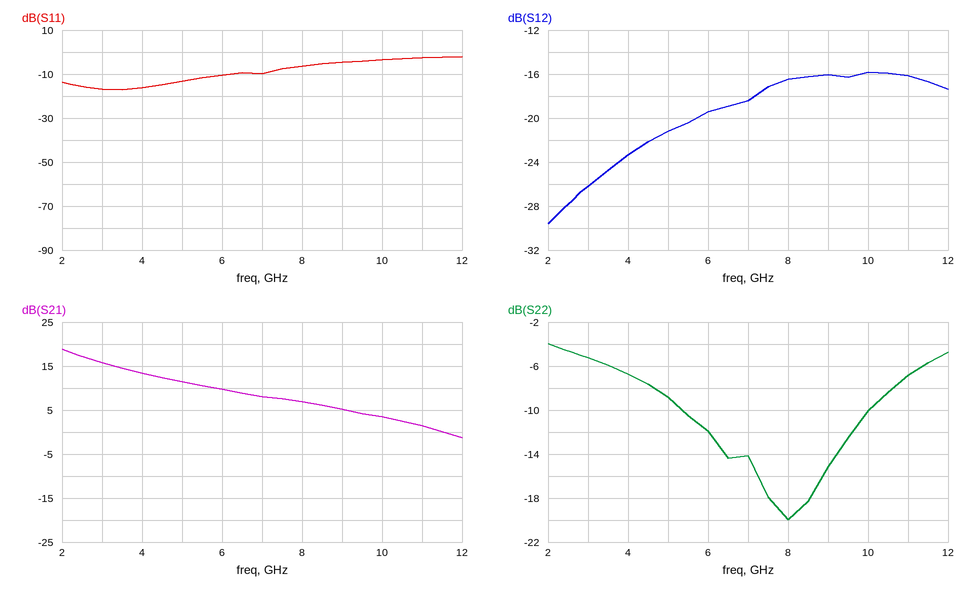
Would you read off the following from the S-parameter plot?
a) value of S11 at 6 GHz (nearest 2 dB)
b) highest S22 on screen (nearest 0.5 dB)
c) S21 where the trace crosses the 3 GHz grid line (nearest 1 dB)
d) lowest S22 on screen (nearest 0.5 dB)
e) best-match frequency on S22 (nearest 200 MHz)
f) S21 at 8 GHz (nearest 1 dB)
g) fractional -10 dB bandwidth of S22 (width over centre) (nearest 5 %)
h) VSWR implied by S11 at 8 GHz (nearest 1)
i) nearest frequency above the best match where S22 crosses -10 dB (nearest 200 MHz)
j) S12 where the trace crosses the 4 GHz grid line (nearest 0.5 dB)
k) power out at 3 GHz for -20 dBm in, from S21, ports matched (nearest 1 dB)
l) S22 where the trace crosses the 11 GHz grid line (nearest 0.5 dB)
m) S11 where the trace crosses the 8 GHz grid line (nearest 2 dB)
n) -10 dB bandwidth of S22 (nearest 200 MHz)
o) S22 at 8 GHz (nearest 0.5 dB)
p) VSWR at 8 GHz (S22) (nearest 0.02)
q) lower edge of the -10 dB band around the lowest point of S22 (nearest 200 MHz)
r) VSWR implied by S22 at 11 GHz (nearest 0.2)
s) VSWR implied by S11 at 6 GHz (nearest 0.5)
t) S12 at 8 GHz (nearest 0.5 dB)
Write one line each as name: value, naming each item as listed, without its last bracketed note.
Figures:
value of S11 at 6 GHz: -10 dB
highest S22 on screen: -4.0 dB
S21 where the trace crosses the 3 GHz grid line: 16 dB
lowest S22 on screen: -20.0 dB
best-match frequency on S22: 8.0 GHz
S21 at 8 GHz: 7 dB
fractional -10 dB bandwidth of S22 (width over centre): 60 %
VSWR implied by S11 at 8 GHz: 3
nearest frequency above the best match where S22 crosses -10 dB: 10.0 GHz
S12 where the trace crosses the 4 GHz grid line: -23.5 dB
power out at 3 GHz for -20 dBm in, from S21, ports matched: -4 dBm
S22 where the trace crosses the 11 GHz grid line: -7.0 dB
S11 where the trace crosses the 8 GHz grid line: -6 dB
-10 dB bandwidth of S22: 4.6 GHz
S22 at 8 GHz: -20.0 dB
VSWR at 8 GHz (S22): 1.22
lower edge of the -10 dB band around the lowest point of S22: 5.4 GHz
VSWR implied by S22 at 11 GHz: 2.6
VSWR implied by S11 at 6 GHz: 2.0
S12 at 8 GHz: -16.5 dB
